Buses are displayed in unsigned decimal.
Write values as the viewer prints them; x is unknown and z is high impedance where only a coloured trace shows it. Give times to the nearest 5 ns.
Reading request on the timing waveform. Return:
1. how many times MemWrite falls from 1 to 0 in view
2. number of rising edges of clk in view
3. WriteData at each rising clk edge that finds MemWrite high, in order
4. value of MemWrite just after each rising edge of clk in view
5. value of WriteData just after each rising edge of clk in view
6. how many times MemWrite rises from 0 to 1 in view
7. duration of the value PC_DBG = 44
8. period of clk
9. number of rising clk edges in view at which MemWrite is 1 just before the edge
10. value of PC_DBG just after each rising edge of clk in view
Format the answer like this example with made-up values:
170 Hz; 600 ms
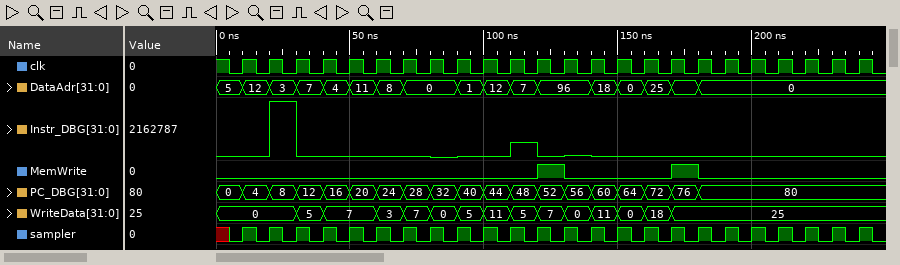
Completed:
2; 24; 7, 25; 0 0 0 0 0 0 0 0 0 0 0 1 0 0 0 0 1 0 0 0 0 0 0 0; 0, 0, 5, 7, 7, 3, 7, 0, 5, 11, 5, 7, 0, 11, 0, 18, 25, 25, 25, 25, 25, 25, 25, 25; 2; 10 ns; 10 ns; 2; 4, 8, 12, 16, 20, 24, 28, 32, 40, 44, 48, 52, 56, 60, 64, 72, 76, 80, 80, 80, 80, 80, 80, 80
